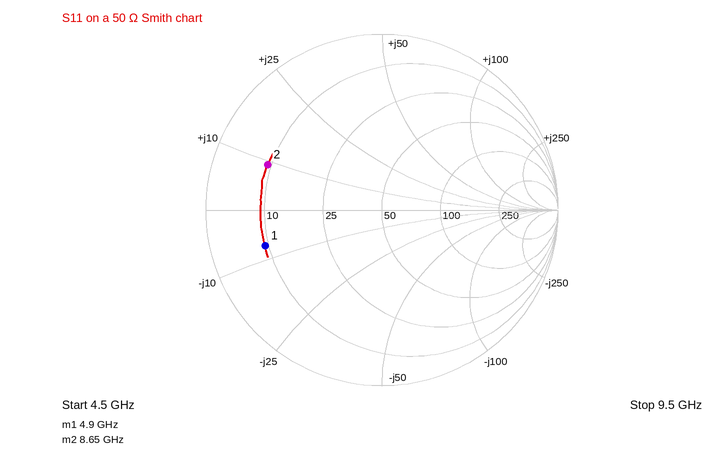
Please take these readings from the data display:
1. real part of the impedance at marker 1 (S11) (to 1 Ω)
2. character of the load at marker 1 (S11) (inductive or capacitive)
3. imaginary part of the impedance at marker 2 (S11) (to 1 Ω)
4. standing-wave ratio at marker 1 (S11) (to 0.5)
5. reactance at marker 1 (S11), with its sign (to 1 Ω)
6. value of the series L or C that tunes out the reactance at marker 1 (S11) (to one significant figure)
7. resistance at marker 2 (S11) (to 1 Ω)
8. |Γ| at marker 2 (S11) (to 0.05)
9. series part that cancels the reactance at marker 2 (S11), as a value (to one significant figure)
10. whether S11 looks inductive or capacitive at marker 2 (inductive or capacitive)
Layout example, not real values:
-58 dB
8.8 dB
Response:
9 Ω
capacitive
+9 Ω
5.5
-7 Ω
200 pH
9 Ω
0.70
2 pF
inductive
